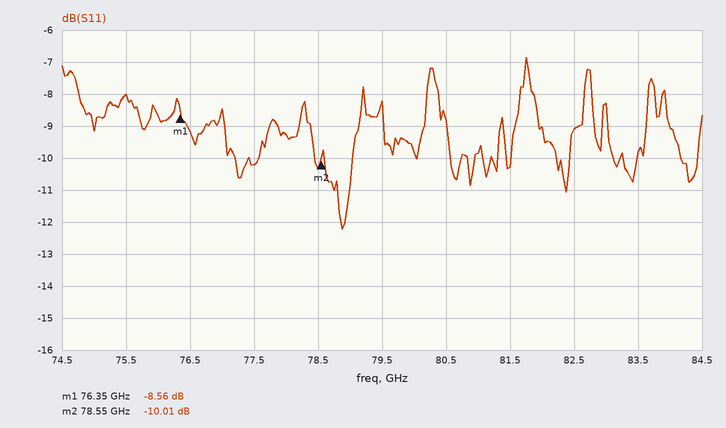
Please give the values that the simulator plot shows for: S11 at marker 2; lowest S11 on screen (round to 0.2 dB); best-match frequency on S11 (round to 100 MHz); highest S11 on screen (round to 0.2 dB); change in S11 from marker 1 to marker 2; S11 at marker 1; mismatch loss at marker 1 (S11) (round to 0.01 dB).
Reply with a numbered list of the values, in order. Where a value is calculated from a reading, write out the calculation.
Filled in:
1. -10.01 dB
2. -12.2 dB
3. 78.9 GHz
4. -6.8 dB
5. -10.01 − (-8.56) = -1.45 dB
6. -8.56 dB
7. −10 log10(1 − 10^(-8.56/10)) ≈ 0.65 dB
